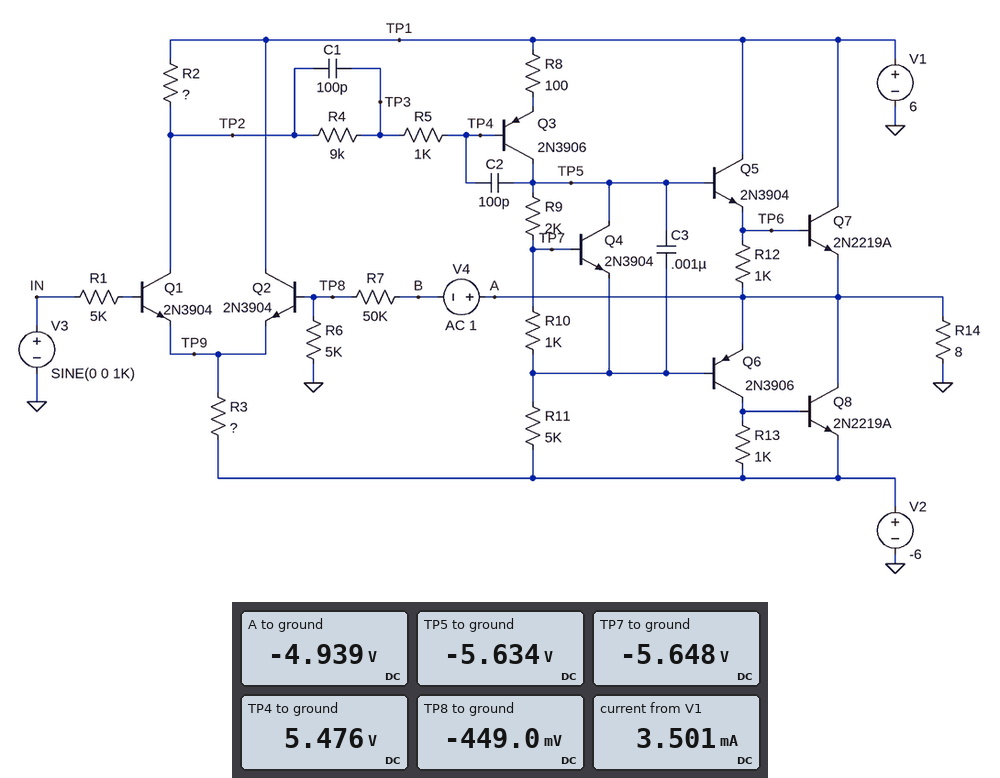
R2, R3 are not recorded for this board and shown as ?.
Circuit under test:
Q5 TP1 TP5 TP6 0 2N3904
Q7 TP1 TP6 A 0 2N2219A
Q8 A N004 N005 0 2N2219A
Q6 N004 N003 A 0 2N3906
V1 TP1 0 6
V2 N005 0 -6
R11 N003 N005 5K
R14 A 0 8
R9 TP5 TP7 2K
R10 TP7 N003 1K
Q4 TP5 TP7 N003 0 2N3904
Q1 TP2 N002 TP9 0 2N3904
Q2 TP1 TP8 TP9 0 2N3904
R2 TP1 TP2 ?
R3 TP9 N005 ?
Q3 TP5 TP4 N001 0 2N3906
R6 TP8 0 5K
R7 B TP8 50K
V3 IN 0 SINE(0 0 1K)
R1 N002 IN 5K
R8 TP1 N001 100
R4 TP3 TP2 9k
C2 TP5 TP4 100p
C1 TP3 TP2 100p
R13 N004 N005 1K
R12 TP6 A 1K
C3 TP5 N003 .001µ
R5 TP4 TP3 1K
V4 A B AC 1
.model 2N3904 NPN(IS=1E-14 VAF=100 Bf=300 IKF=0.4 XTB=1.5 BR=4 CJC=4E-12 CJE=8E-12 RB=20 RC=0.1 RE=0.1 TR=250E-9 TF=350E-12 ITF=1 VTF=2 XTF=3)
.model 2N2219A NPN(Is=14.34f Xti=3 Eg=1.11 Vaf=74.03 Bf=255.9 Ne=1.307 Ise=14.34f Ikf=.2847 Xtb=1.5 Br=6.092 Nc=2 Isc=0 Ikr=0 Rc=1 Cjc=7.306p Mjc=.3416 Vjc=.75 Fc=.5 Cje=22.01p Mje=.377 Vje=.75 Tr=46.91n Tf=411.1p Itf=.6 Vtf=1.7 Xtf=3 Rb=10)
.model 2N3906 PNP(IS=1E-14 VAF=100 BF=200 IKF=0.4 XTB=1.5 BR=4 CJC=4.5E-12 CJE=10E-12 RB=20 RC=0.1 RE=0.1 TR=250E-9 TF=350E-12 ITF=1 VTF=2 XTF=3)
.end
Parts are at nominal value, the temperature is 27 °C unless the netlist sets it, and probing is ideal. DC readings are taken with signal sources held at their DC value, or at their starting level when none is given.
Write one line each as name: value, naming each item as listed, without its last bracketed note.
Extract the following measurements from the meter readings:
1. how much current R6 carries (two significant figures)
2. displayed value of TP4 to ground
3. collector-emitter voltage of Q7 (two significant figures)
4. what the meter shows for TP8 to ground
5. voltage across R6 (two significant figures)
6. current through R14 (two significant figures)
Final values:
how much current R6 carries: 90 µA
displayed value of TP4 to ground: 5.476 V
collector-emitter voltage of Q7: 11 V
what the meter shows for TP8 to ground: -449.0 mV
voltage across R6: 450 mV
current through R14: 620 mA
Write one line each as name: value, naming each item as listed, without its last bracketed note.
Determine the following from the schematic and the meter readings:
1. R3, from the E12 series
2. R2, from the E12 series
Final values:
R3, from the E12 series: 1.5 kΩ
R2, from the E12 series: 150 Ω
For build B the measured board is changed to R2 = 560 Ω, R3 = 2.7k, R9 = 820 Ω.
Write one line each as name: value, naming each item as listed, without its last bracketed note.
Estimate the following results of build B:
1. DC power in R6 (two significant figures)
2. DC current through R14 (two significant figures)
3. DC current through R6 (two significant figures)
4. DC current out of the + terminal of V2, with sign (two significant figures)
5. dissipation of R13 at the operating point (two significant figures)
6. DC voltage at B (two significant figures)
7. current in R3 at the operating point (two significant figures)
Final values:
DC power in R6: 470 nW
DC current through R14: 56 mA
DC current through R6: 9.7 µA
DC current out of the + terminal of V2, with sign: -59 mA
dissipation of R13 at the operating point: 570 µW
DC voltage at B: -450 mV
current in R3 at the operating point: 2.0 mA
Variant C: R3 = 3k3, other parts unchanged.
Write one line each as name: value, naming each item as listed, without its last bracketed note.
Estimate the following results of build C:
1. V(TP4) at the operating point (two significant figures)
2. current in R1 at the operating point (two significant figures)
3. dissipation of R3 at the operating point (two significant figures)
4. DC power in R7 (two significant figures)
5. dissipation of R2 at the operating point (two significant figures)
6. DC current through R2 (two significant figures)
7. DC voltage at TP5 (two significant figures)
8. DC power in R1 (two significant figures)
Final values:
V(TP4) at the operating point: 5.8 V
current in R1 at the operating point: 5.1 µA
dissipation of R3 at the operating point: 8.5 mW
DC power in R7: 400 µW
dissipation of R2 at the operating point: 390 µW
DC current through R2: 1.6 mA
DC voltage at TP5: -5.7 V
DC power in R1: 130 nW
